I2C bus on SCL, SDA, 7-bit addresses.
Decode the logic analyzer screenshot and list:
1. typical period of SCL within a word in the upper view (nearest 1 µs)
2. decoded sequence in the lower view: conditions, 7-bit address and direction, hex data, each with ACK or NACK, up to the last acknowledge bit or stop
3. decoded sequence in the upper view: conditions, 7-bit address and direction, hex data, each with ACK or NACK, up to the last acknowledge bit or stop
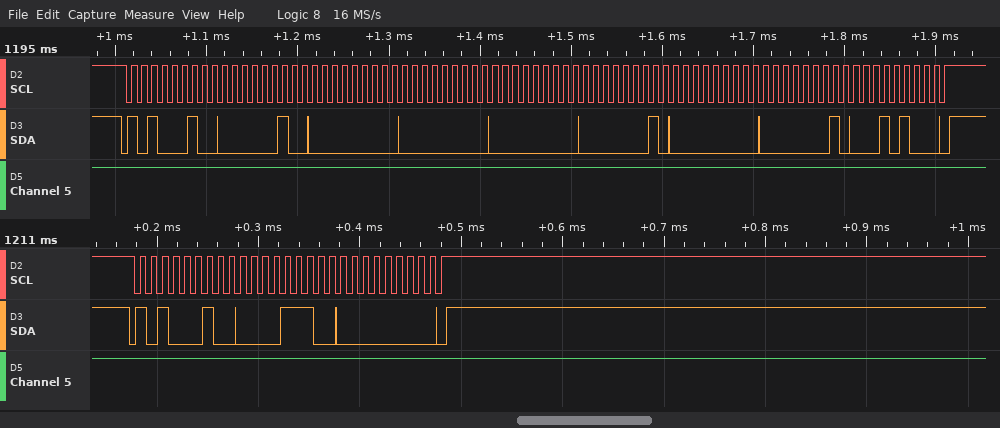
11 µs
start, address 51 write ACK, 0E ACK, 00 ACK, stop
start, address 51 write ACK, 02 ACK, 00 ACK, 00 ACK, 00 ACK, 01 ACK, 00 ACK, 01 ACK, 14 ACK, stop
